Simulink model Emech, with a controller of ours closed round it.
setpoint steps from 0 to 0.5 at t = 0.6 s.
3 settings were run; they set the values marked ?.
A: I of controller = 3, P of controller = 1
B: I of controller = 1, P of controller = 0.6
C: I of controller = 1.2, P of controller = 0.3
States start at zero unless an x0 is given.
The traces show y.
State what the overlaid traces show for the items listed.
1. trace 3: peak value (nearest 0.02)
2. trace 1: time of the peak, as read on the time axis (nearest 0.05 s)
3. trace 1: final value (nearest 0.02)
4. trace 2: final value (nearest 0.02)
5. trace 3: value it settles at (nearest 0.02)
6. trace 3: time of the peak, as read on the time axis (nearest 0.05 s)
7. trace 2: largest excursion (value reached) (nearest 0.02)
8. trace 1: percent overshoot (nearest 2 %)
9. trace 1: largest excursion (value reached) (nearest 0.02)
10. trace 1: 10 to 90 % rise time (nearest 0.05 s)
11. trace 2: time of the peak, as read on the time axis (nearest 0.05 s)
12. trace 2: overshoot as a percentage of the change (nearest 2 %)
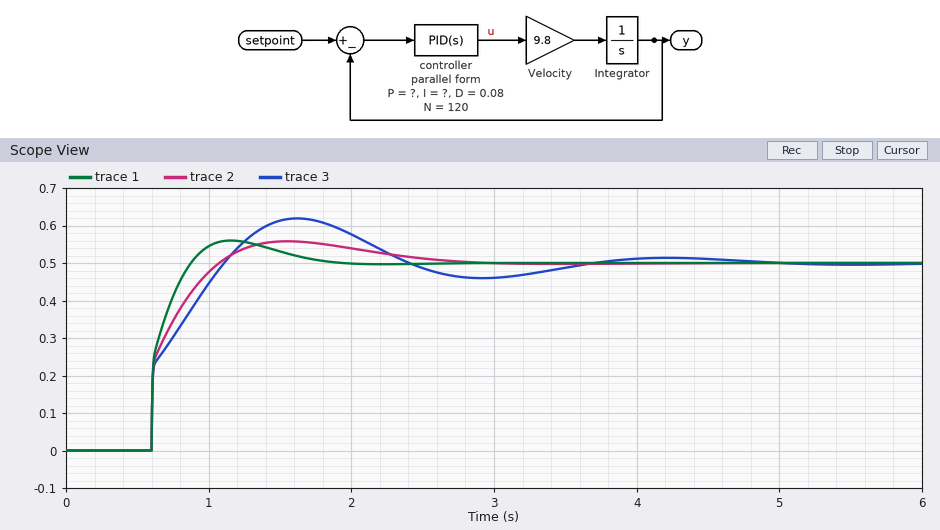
0.62
1.15 s
0.50
0.50
0.50
1.60 s
0.56
12 %
0.56
0.20 s
1.55 s
12 %
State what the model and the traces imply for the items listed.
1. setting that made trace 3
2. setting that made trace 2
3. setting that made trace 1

C
B
A
